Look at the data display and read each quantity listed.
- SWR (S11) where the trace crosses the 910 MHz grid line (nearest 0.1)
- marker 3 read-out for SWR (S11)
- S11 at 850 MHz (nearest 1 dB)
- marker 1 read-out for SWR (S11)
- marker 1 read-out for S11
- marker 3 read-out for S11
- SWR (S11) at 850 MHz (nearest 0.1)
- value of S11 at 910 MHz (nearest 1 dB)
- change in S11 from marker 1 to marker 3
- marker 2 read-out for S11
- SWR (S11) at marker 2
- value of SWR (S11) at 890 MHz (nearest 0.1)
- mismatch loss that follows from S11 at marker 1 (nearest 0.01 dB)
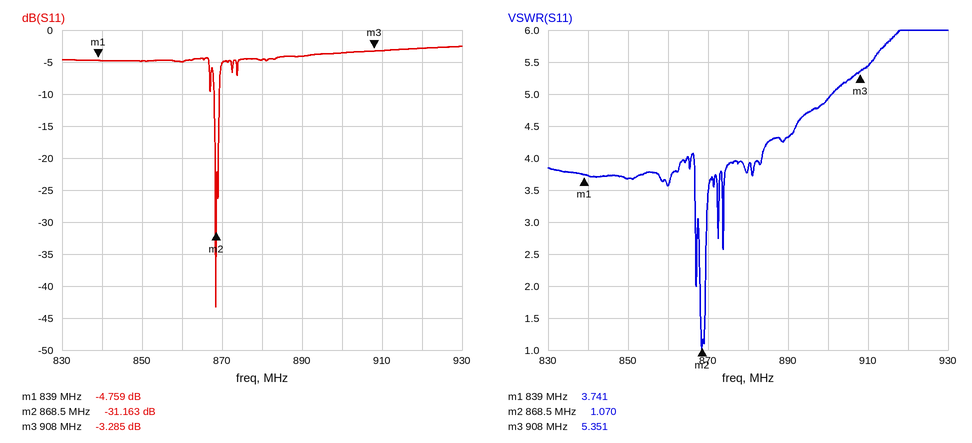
5.4
5.351
-5 dB
3.741
-4.759 dB
-3.285 dB
3.7
-3 dB
1.474 dB
-31.163 dB
1.070
4.3
1.77 dB
